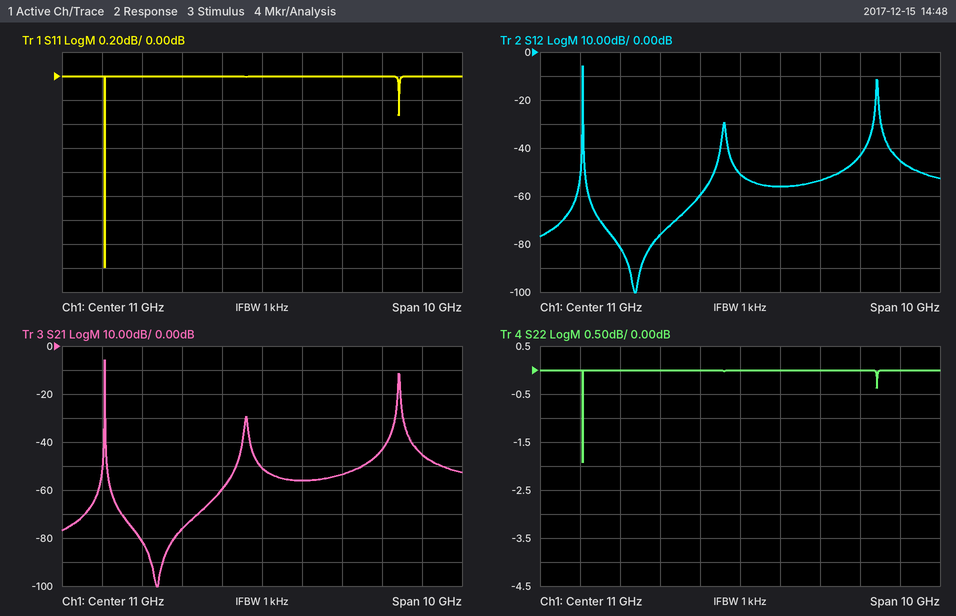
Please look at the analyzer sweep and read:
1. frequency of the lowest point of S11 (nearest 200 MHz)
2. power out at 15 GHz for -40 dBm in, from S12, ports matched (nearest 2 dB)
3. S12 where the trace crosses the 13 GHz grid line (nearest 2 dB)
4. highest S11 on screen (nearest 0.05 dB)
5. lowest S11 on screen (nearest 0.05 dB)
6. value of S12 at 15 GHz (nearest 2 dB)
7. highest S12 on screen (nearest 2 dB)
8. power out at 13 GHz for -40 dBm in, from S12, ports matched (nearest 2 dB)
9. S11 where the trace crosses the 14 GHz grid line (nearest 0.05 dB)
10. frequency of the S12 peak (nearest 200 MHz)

7.0 GHz
-86 dBm
-54 dB
0.00 dB
-1.60 dB
-46 dB
-6 dB
-94 dBm
0.00 dB
7.0 GHz
